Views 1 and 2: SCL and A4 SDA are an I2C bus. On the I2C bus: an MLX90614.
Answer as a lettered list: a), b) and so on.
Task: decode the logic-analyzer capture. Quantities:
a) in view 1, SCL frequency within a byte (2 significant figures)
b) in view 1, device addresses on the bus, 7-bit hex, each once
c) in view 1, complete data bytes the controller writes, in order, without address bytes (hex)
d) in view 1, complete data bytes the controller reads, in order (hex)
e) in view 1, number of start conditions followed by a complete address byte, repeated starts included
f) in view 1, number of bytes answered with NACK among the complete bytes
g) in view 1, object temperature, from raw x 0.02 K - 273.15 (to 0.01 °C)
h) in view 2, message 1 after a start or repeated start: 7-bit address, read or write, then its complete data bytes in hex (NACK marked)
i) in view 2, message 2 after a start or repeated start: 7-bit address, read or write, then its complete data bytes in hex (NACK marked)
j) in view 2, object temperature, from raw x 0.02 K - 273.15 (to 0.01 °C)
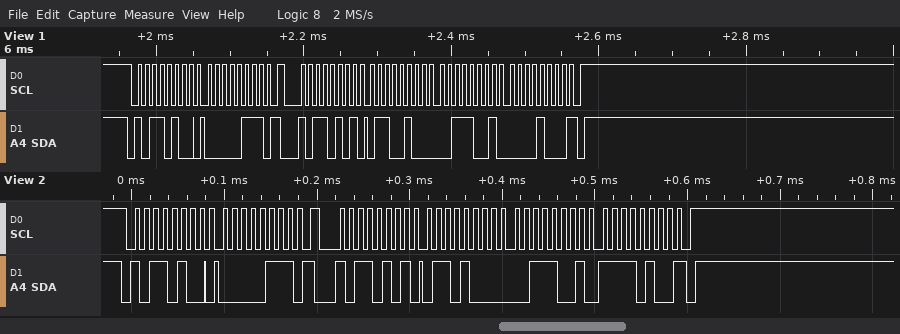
a) 100 kHz
b) 0x5A
c) 07
d) 64 39 08
e) 2
f) 1
g) 20.69 °C
h) 0x5A write: 07
i) 0x5A read: 68 39 F4 NACK
j) 20.77 °C
